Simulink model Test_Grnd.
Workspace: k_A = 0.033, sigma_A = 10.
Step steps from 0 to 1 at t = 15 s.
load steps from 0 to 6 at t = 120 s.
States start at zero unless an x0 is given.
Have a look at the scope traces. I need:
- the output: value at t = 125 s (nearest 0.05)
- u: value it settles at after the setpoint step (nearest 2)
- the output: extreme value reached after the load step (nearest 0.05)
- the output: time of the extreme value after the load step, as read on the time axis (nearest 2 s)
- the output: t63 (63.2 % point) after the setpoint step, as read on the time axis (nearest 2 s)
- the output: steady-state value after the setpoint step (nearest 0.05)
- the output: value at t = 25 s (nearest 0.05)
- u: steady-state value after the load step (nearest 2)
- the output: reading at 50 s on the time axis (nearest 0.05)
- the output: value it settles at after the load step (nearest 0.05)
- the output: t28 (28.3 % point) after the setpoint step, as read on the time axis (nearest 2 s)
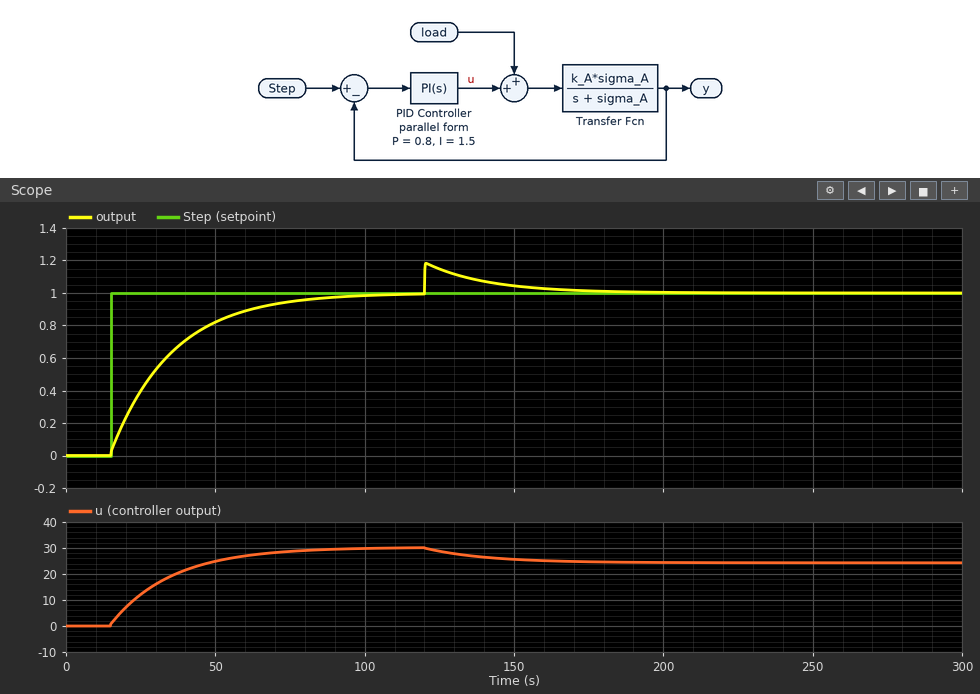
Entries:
1.15
30
1.20
120 s
36 s
1.00
0.40
24
0.80
1.00
22 s
